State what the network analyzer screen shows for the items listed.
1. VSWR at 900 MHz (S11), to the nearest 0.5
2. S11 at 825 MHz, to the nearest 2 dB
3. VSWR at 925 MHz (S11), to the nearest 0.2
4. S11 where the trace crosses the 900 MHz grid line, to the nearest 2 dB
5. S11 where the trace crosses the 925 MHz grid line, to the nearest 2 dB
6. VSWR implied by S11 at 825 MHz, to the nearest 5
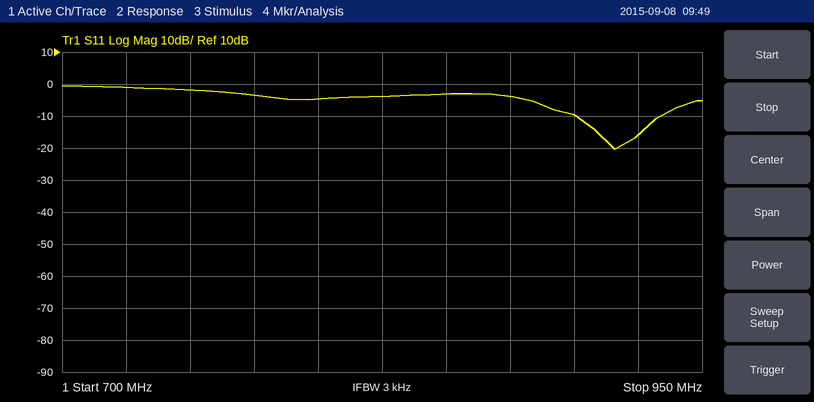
2.0
-4 dB
1.4
-10 dB
-16 dB
5
